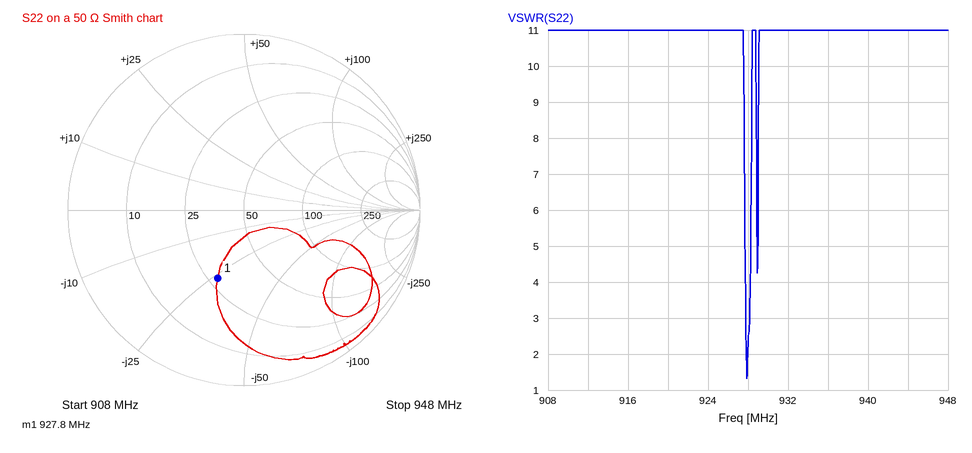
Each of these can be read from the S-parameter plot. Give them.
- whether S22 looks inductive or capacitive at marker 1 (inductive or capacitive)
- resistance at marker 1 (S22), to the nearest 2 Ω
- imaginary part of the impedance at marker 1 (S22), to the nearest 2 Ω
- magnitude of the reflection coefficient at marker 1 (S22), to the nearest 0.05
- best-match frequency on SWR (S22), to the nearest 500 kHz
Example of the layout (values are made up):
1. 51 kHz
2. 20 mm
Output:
1. capacitive
2. 28 Ω
3. -26 Ω
4. 0.40
5. 928.0 MHz
